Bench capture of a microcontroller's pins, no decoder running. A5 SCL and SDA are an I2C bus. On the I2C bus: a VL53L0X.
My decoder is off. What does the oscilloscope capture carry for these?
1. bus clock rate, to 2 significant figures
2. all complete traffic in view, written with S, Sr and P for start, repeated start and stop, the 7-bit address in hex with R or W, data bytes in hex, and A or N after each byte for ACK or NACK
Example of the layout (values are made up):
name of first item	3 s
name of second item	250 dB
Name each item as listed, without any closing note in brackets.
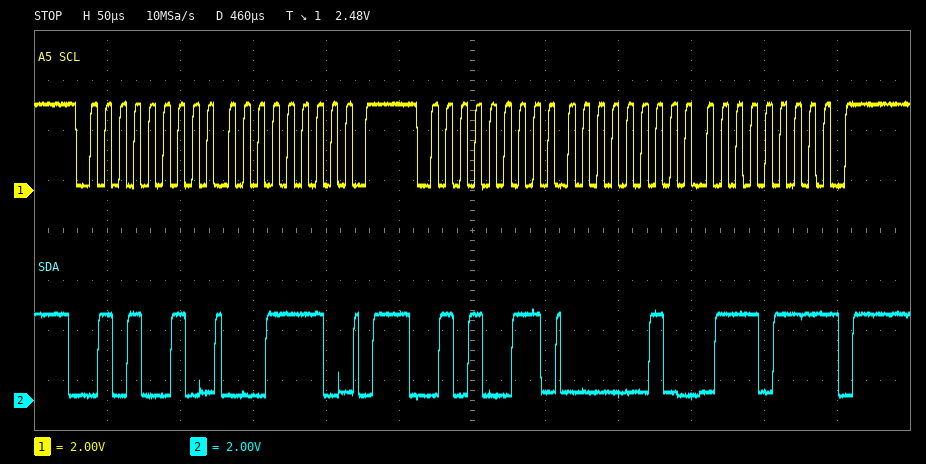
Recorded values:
bus clock rate, to 2 significant figures	100 kHz
all complete traffic in view, written with S, Sr and P for start, repeated start and stop, the 7-bit address in hex with R or W, data bytes in hex, and A or N after each byte for ACK or NACK	S 29W A 1E A P S 29R A 02 A 77 N P
